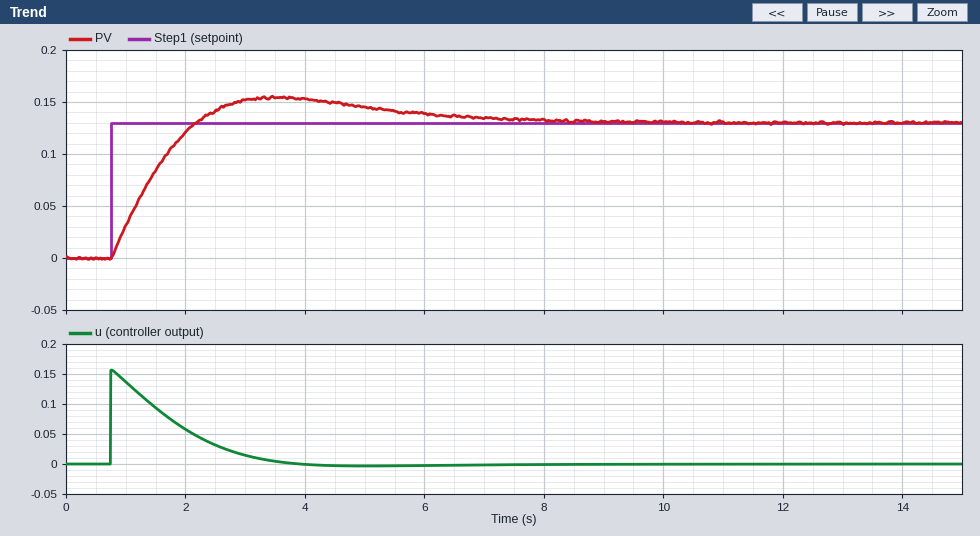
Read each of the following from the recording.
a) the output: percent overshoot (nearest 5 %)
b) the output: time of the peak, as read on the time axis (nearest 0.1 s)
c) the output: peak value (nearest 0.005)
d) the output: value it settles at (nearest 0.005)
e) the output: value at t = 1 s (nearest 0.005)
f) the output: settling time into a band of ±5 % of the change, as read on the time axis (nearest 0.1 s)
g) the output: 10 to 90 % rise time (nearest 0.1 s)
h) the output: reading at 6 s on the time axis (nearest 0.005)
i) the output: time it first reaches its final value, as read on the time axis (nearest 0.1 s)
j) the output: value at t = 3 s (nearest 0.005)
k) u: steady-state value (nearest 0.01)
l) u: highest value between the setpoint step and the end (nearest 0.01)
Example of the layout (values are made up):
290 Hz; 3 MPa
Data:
20 %; 3.5 s; 0.155; 0.130; 0.030; 6.5 s; 1.1 s; 0.140; 2.2 s; 0.150; 0.00; 0.16
